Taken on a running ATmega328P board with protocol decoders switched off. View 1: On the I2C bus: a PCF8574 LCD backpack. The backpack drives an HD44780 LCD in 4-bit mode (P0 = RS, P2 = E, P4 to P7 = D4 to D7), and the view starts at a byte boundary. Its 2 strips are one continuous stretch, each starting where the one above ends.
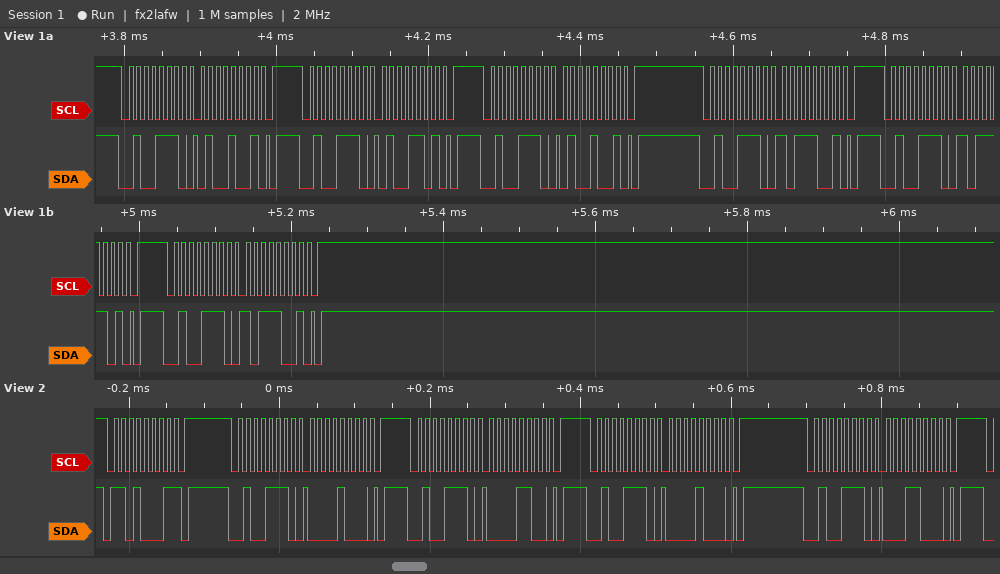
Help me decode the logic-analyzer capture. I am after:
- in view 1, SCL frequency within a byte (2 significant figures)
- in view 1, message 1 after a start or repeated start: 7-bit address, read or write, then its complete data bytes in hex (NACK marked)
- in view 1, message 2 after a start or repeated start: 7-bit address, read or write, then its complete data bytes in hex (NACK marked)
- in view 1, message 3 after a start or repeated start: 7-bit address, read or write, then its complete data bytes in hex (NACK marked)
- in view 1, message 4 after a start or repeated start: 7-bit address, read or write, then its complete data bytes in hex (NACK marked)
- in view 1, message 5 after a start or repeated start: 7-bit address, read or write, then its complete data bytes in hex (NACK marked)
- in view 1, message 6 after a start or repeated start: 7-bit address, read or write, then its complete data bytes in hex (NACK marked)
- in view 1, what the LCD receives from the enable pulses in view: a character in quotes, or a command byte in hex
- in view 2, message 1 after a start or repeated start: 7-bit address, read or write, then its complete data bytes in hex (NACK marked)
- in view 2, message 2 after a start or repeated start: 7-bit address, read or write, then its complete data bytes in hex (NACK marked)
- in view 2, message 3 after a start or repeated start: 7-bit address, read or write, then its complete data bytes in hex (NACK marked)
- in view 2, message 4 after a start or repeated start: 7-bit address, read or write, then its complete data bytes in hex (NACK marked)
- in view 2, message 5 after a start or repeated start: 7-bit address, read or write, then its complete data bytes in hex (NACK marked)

100 kHz
0x27 write: 49
0x27 write: 4D
0x27 write: 49
0x27 write: B9
0x27 write: BD
0x27 write: B9
'K'
0x68 read NACK
0x27 write: 08
0x27 write: 0C
0x27 write: 08
0x27 write: 18
